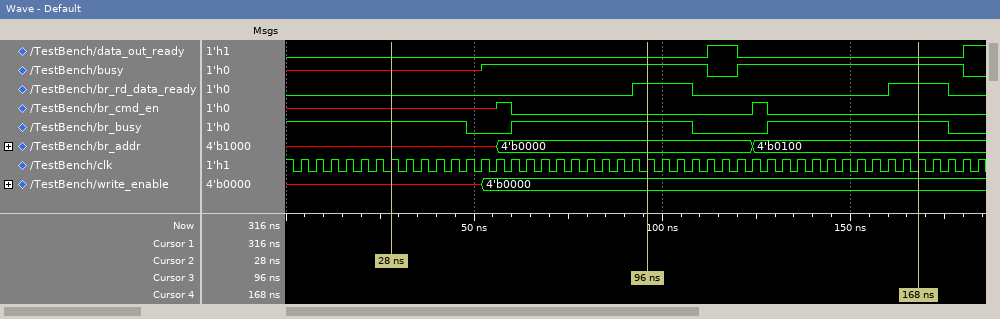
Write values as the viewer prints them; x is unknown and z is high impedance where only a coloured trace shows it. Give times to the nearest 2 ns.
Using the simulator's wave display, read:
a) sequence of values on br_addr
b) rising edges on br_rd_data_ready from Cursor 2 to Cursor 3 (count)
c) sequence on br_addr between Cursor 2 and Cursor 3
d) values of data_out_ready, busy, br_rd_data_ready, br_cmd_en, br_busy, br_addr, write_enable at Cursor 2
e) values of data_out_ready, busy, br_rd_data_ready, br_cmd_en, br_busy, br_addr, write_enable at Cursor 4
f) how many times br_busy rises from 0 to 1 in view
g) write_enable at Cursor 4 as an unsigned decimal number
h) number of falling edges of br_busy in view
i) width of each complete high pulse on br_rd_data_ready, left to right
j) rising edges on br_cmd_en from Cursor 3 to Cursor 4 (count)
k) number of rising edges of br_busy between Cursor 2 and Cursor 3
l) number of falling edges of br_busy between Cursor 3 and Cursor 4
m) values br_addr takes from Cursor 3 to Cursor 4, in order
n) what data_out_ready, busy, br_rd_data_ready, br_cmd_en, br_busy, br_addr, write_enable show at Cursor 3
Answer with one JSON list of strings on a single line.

["x, 4'b0000, 4'b0100", "1", "x, 4'b0000", "data_out_ready=0, busy=x, br_rd_data_ready=0, br_cmd_en=x, br_busy=1, br_addr=x, write_enable=x", "data_out_ready=0, busy=1, br_rd_data_ready=1, br_cmd_en=0, br_busy=1, br_addr=4'b0100, write_enable=4'b0000", "2", "0", "3", "16 ns, 16 ns", "1", "1", "1", "4'b0000, 4'b0100", "data_out_ready=0, busy=1, br_rd_data_ready=1, br_cmd_en=0, br_busy=1, br_addr=4'b0000, write_enable=4'b0000"]
